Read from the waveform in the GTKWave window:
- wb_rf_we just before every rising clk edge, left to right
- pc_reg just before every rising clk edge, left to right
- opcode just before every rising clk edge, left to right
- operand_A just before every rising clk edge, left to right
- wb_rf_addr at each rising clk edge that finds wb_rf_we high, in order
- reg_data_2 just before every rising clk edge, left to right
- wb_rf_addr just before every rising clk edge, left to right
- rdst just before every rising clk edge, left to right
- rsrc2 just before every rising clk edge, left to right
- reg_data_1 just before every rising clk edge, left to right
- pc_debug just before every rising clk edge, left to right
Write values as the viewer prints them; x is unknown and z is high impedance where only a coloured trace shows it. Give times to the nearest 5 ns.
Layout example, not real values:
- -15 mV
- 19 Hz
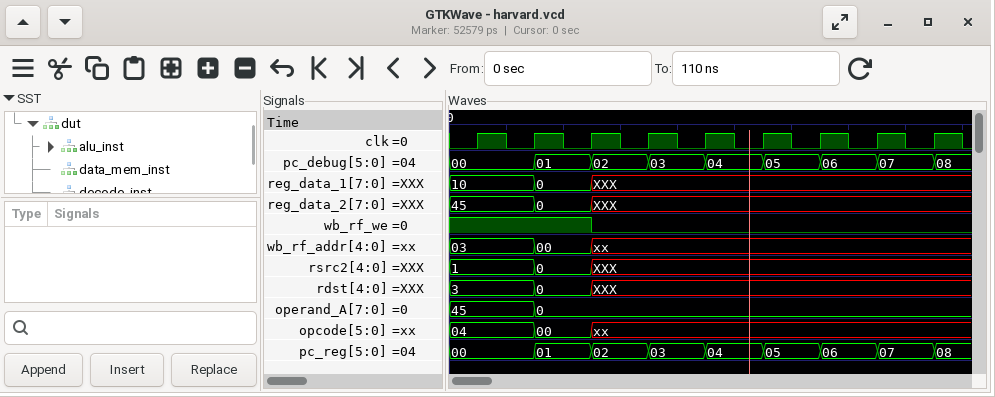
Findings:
- 1 1 1 0 0 0 0 0 0
- 00, 00, 01, 02, 03, 04, 05, 06, 07
- 04, 04, 00, xx, xx, xx, xx, xx, xx
- 45, 45, 0, 0, 0, 0, 0, 0, 0
- 03, 03, 00
- 45, 45, 0, XXX, XXX, XXX, XXX, XXX, XXX
- 03, 03, 00, xx, xx, xx, xx, xx, xx
- 3, 3, 0, XXX, XXX, XXX, XXX, XXX, XXX
- 1, 1, 0, XXX, XXX, XXX, XXX, XXX, XXX
- 10, 10, 0, XXX, XXX, XXX, XXX, XXX, XXX
- 00, 00, 01, 02, 03, 04, 05, 06, 07
